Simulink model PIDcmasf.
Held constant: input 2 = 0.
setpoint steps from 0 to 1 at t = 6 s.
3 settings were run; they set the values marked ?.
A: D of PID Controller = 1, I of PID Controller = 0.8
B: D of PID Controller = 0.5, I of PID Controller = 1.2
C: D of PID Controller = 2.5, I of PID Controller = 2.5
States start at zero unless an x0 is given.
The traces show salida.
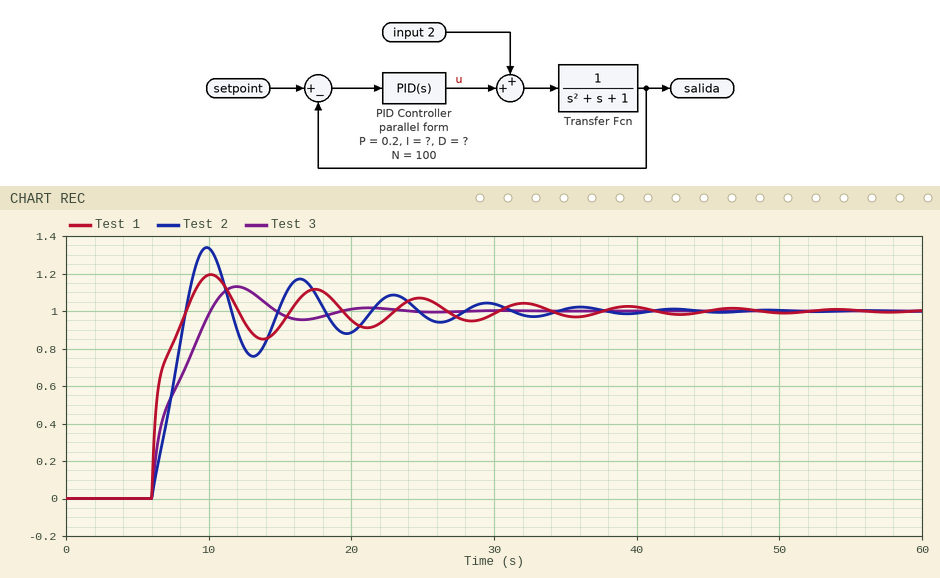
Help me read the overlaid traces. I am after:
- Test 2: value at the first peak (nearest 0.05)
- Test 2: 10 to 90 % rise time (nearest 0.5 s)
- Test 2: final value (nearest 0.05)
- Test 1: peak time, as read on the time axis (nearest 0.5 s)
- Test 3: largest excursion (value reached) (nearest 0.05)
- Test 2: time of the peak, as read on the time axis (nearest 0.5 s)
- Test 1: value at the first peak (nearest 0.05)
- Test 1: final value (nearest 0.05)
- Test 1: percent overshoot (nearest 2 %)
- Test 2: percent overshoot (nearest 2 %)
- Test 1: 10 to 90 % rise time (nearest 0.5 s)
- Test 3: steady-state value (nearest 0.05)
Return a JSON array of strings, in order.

["1.35", "2.0 s", "1.00", "10.0 s", "1.15", "10.0 s", "1.20", "1.00", "20 %", "34 %", "2.0 s", "1.00"]
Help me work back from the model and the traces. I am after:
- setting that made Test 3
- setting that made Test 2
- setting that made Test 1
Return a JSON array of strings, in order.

["A", "B", "C"]
